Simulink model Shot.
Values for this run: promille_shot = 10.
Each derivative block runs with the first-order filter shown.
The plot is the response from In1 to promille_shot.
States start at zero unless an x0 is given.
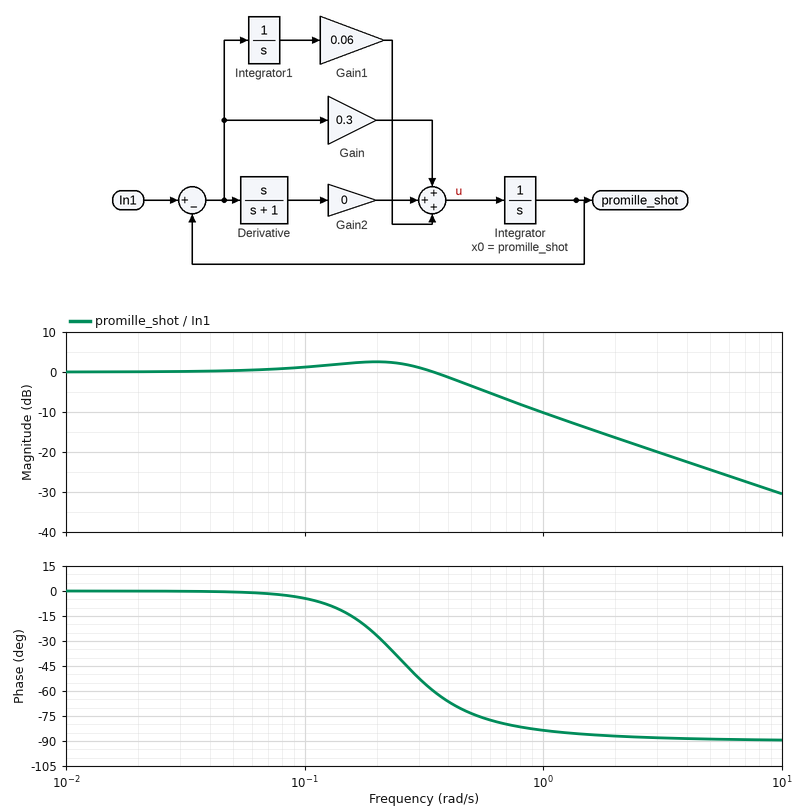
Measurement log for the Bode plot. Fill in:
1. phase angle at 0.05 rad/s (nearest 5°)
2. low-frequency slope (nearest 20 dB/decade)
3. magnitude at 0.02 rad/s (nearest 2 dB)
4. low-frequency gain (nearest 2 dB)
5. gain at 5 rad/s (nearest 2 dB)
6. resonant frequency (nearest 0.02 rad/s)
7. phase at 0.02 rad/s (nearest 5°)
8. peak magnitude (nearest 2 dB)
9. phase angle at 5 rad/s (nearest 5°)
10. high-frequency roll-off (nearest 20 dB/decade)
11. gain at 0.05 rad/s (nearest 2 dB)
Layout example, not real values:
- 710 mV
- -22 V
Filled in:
- 0°
- 0 dB/decade
- 0 dB
- 0 dB
- -24 dB
- 0.20 rad/s
- 0°
- 2 dB
- -90°
- -20 dB/decade
- 0 dB
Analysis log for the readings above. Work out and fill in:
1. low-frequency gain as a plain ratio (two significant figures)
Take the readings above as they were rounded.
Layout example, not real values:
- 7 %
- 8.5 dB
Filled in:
- 1.0
